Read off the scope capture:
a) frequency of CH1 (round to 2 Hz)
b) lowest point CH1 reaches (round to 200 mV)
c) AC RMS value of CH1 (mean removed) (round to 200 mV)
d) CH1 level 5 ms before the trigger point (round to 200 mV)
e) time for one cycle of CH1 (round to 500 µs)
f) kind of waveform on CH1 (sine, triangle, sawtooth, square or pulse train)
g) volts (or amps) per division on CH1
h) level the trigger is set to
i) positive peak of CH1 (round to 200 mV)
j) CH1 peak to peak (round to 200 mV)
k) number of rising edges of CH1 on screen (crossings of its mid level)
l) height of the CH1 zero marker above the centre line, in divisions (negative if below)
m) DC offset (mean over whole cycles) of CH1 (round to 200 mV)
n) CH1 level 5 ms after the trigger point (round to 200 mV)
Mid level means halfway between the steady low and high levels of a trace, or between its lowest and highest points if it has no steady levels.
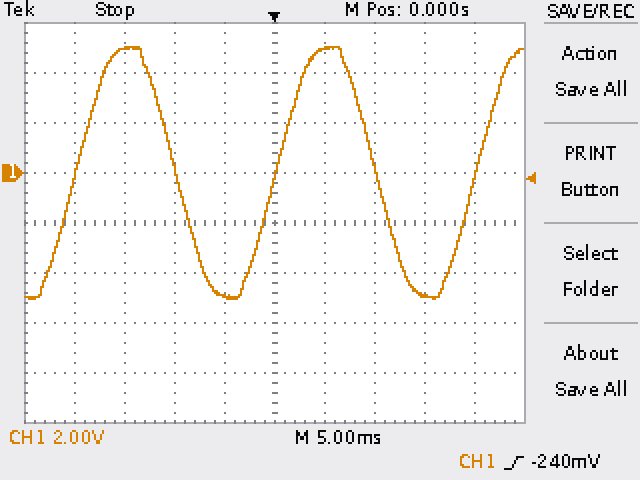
50 Hz
-5.0 V
3.6 V
-5.0 V
20.0 ms
sine
2 V
-240 mV
5.0 V
10.0 V
3
+1.0 div
0.0 V
5.0 V
